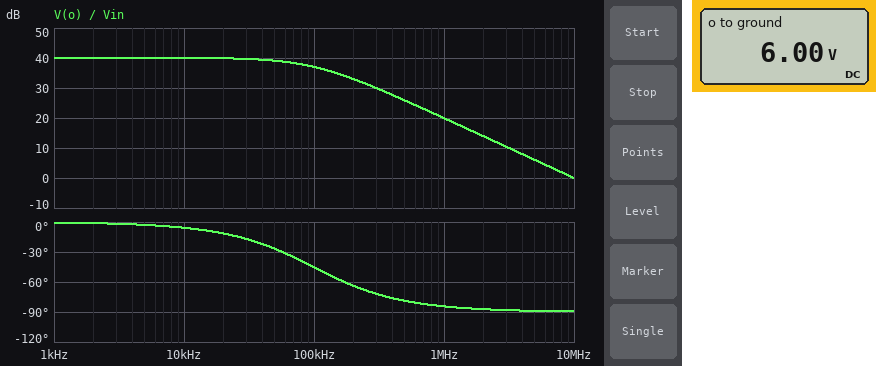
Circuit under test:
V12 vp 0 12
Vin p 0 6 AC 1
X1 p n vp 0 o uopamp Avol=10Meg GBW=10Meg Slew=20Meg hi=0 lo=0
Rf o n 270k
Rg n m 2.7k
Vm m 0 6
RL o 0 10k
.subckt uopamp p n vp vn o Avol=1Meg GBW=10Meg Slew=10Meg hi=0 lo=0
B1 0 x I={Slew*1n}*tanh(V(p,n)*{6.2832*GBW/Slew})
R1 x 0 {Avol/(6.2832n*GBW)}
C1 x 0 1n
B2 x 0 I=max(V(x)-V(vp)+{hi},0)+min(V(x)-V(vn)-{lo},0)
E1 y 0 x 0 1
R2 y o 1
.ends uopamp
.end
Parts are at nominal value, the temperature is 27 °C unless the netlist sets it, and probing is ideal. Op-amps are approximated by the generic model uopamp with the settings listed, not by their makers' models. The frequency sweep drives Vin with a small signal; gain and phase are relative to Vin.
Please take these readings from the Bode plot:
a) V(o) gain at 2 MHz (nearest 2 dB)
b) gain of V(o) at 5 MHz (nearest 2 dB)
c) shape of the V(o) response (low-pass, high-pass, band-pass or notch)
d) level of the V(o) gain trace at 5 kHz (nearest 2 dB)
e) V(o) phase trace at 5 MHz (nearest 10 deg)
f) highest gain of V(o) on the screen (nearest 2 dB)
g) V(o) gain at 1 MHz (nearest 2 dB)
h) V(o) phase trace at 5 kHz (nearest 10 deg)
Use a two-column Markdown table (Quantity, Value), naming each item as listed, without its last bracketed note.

| Quantity | Value |
|---|---|
| V(o) gain at 2 MHz | 14 dB |
| gain of V(o) at 5 MHz | 6 dB |
| shape of the V(o) response | low-pass |
| level of the V(o) gain trace at 5 kHz | 40 dB |
| V(o) phase trace at 5 MHz | -90 deg |
| highest gain of V(o) on the screen | 40 dB |
| V(o) gain at 1 MHz | 20 dB |
| V(o) phase trace at 5 kHz | 0 deg |
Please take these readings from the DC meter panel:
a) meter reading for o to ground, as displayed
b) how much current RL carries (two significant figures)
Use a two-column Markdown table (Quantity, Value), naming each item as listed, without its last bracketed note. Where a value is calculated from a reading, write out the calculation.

| Quantity | Value |
|---|---|
| meter reading for o to ground, as displayed | 6.00 V |
| how much current RL carries | (6 V) / 10 kΩ = 600 µA |
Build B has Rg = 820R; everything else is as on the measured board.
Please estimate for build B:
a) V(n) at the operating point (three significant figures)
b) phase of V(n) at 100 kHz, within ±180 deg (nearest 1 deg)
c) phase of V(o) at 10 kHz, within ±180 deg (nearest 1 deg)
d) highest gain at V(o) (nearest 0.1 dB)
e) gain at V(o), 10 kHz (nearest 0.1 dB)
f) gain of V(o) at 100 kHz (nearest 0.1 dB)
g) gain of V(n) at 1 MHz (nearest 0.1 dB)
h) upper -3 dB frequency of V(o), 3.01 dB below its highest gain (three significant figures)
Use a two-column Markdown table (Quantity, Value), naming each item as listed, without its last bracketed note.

| Quantity | Value |
|---|---|
| V(n) at the operating point | 6.00 V |
| phase of V(n) at 100 kHz, within ±180 deg | -73 deg |
| phase of V(o) at 10 kHz, within ±180 deg | -18 deg |
| highest gain at V(o) | 50.4 dB |
| gain at V(o), 10 kHz | 49.9 dB |
| gain of V(o) at 100 kHz | 39.6 dB |
| gain of V(n) at 1 MHz | -30.4 dB |
| upper -3 dB frequency of V(o), 3.01 dB below its highest gain | 30.3 kHz |
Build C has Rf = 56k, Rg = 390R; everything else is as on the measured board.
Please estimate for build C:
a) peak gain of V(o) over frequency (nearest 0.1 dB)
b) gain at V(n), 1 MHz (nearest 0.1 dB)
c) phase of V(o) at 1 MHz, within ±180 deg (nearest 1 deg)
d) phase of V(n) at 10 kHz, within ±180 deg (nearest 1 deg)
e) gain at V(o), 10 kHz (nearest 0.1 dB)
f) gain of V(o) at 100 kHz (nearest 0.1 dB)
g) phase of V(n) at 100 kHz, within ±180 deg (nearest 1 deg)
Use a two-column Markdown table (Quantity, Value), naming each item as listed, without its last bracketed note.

| Quantity | Value |
|---|---|
| peak gain of V(o) over frequency | 43.2 dB |
| gain at V(n), 1 MHz | -23.2 dB |
| phase of V(o) at 1 MHz, within ±180 deg | -86 deg |
| phase of V(n) at 10 kHz, within ±180 deg | -8 deg |
| gain at V(o), 10 kHz | 43.1 dB |
| gain of V(o) at 100 kHz | 38.3 dB |
| phase of V(n) at 100 kHz, within ±180 deg | -55 deg |
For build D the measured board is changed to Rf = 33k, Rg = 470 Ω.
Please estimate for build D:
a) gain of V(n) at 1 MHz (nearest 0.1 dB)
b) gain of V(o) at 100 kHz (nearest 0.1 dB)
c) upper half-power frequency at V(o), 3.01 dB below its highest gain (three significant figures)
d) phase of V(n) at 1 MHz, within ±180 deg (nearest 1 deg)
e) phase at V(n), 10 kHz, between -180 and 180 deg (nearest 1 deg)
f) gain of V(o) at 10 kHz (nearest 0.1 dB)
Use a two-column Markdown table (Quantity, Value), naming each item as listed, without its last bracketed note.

| Quantity | Value |
|---|---|
| gain of V(n) at 1 MHz | -17.1 dB |
| gain of V(o) at 100 kHz | 35.3 dB |
| upper half-power frequency at V(o), 3.01 dB below its highest gain | 140 kHz |
| phase of V(n) at 1 MHz, within ±180 deg | -82 deg |
| phase at V(n), 10 kHz, between -180 and 180 deg | -4 deg |
| gain of V(o) at 10 kHz | 37.0 dB |
